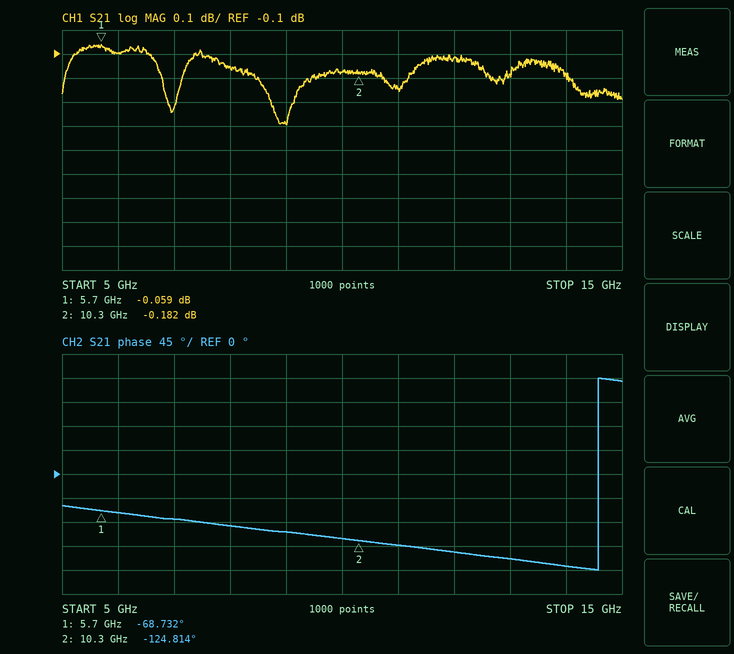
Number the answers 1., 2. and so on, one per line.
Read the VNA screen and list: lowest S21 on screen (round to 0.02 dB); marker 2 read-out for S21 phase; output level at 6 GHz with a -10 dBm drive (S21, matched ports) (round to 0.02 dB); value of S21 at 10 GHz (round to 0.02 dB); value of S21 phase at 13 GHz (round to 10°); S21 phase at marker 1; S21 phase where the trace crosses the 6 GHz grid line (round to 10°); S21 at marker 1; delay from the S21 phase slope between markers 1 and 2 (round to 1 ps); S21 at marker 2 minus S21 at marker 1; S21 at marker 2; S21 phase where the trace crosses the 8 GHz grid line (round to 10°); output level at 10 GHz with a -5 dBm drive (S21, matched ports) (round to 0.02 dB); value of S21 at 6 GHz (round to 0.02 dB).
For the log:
1. -0.40 dB
2. -124.814°
3. -10.10 dBm
4. -0.18 dB
5. -160°
6. -68.732°
7. -70°
8. -0.059 dB
9. 34 ps
10. -0.123 dB
11. -0.182 dB
12. -100°
13. -5.18 dBm
14. -0.10 dB
